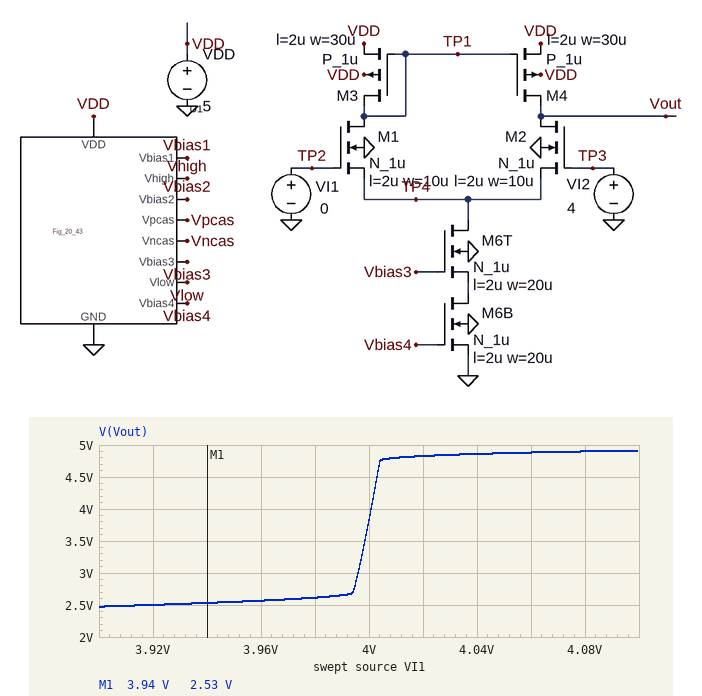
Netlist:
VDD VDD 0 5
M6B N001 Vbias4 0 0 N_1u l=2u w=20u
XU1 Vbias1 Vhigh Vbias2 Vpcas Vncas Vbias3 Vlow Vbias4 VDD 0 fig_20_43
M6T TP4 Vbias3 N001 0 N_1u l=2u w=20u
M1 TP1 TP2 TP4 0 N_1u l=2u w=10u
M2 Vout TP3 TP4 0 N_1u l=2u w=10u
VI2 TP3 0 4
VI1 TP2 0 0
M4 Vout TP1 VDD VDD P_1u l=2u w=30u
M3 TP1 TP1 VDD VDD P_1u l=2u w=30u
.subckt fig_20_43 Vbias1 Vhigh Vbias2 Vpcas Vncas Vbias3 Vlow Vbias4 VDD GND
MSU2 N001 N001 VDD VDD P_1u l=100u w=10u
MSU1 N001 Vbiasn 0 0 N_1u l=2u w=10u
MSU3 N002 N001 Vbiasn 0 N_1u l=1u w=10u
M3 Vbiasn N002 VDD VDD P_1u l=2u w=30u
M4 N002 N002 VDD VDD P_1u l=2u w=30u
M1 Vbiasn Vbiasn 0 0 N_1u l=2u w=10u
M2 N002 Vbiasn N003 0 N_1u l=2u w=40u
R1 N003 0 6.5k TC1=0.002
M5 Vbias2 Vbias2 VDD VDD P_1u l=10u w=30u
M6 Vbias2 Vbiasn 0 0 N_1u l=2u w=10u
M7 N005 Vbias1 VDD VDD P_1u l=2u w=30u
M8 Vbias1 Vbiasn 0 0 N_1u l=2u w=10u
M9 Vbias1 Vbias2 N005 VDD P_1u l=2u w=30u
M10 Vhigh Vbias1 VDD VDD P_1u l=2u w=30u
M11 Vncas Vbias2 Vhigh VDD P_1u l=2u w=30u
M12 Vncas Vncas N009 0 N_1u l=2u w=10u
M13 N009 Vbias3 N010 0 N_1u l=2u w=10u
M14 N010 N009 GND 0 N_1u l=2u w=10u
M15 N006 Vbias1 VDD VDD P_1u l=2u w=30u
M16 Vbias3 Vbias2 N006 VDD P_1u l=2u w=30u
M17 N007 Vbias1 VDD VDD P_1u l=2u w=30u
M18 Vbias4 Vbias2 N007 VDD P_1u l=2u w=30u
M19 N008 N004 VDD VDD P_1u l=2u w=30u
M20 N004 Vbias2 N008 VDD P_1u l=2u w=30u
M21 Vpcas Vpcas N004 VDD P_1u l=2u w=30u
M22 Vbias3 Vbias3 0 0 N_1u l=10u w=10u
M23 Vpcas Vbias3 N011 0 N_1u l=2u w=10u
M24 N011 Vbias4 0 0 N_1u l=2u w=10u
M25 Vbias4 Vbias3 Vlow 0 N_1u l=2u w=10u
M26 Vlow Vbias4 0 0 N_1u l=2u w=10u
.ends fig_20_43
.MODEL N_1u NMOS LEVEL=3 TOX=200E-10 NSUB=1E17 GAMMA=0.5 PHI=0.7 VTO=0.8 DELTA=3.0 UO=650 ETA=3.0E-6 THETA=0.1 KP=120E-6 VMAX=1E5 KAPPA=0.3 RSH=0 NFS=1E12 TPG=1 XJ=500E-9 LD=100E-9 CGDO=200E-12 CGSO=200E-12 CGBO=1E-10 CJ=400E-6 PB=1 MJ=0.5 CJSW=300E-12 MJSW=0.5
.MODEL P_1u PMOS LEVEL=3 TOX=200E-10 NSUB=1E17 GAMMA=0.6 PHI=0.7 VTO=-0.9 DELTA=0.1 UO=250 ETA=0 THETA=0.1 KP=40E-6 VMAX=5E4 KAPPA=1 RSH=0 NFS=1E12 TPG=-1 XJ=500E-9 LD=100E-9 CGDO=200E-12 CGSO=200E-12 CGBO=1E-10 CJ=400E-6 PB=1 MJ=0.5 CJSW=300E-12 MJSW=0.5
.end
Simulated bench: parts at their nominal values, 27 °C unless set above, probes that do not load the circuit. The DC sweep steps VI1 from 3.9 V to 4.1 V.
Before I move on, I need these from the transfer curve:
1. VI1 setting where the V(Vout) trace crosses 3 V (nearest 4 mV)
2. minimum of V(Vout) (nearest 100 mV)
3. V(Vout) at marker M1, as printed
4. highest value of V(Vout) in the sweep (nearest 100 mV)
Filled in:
3.996 V
2.5 V
2.53 V
4.9 V
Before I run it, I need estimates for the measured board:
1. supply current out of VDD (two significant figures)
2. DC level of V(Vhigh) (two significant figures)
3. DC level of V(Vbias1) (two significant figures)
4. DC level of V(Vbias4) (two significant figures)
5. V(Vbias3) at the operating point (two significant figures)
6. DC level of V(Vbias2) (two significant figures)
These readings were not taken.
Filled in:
190 µA
4.7 V
3.8 V
1.1 V
1.5 V
3.4 V
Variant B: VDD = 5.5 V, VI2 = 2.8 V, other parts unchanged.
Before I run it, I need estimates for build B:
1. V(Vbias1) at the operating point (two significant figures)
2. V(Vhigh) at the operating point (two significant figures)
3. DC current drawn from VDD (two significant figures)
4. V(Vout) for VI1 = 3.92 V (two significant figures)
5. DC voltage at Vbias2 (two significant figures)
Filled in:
4.3 V
5.2 V
200 µA
5.5 V
3.9 V
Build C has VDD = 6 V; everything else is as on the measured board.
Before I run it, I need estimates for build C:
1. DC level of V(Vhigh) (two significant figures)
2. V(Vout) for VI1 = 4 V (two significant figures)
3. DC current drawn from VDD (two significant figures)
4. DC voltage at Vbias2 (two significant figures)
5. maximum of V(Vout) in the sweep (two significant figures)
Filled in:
5.7 V
4.8 V
200 µA
4.4 V
5.9 V
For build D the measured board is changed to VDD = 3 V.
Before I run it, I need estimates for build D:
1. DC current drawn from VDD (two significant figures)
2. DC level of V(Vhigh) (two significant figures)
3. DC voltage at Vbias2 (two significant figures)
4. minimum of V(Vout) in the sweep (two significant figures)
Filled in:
160 µA
2.7 V
1.5 V
1.8 V
